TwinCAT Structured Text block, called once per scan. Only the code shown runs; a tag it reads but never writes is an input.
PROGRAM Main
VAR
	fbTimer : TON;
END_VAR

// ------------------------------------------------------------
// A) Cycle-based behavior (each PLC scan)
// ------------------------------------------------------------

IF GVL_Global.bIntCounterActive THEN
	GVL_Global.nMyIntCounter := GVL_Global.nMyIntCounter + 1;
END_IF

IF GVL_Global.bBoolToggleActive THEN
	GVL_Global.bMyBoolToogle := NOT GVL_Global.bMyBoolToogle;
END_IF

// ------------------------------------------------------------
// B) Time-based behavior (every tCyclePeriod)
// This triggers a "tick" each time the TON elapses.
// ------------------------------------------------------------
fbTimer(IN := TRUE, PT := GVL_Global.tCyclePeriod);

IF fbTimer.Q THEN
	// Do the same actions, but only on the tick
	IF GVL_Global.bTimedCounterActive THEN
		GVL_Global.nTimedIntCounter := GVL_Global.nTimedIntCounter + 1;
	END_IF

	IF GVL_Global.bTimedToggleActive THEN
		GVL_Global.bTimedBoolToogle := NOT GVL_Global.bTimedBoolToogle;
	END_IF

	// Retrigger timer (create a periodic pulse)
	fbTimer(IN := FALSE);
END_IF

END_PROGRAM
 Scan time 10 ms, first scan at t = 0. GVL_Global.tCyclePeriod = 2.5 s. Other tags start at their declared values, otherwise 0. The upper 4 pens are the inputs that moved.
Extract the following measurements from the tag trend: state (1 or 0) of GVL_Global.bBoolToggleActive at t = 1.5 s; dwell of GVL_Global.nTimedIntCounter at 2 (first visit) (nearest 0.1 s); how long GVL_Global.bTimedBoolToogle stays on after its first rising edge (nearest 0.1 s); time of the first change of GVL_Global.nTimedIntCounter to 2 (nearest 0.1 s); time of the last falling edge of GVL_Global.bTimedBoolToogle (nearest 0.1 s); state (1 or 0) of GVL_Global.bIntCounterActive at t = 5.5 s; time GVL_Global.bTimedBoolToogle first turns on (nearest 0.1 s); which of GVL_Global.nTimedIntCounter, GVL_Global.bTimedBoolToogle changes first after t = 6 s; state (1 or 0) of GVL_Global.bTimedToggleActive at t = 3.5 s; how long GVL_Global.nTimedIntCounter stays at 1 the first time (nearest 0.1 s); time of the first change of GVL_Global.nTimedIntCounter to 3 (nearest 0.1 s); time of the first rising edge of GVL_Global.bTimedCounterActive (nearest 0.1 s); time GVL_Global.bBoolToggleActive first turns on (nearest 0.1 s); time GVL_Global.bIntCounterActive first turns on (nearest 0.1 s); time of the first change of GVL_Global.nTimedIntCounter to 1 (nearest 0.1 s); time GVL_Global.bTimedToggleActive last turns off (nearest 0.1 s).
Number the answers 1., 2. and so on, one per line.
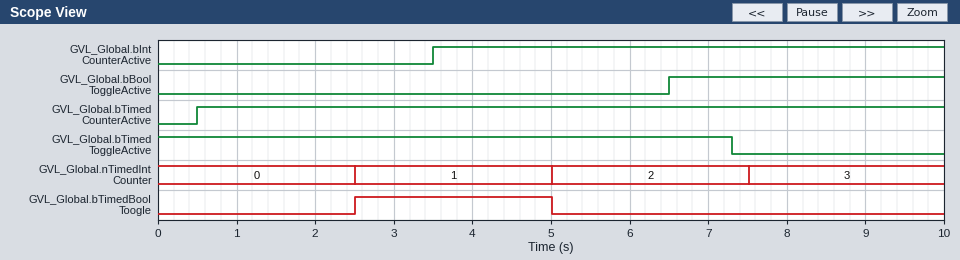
1. 0
2. 2.5 s
3. 2.5 s
4. 5.0 s
5. 5.0 s
6. 1
7. 2.5 s
8. GVL_Global.nTimedIntCounter
9. 1
10. 2.5 s
11. 7.5 s
12. 0.5 s
13. 6.5 s
14. 3.5 s
15. 2.5 s
16. 7.3 s
